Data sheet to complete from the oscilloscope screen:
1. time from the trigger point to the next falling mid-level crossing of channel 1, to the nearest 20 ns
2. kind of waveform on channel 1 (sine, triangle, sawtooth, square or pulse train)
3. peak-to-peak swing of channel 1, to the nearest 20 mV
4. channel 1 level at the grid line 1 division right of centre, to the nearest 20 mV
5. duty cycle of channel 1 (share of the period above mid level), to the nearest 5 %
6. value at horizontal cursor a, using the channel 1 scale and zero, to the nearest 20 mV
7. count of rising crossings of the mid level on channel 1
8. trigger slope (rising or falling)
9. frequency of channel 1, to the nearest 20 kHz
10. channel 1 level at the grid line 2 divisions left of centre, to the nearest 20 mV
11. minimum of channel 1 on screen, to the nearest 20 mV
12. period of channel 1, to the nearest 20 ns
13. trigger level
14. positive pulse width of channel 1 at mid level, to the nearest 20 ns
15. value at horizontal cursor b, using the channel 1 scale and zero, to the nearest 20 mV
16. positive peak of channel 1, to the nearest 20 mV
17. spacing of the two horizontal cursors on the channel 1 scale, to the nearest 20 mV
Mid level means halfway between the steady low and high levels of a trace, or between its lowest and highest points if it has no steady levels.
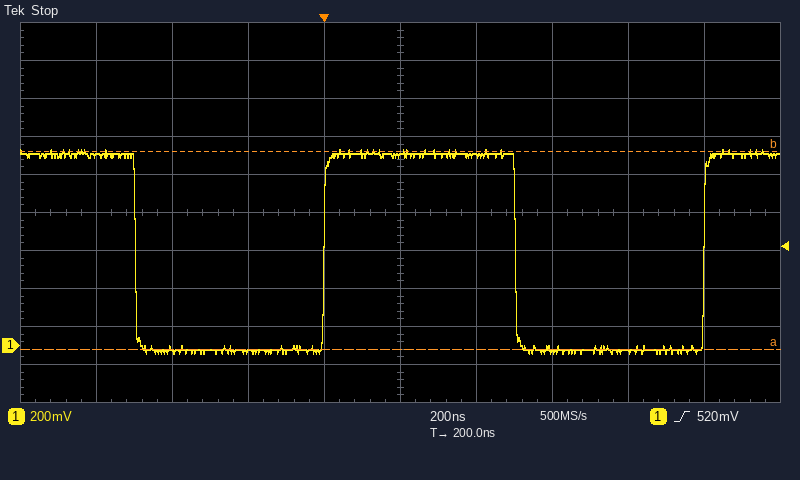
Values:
500 ns
square
1.08 V
1.00 V
50 %
-20 mV
2
rising
1.00 MHz
-40 mV
-40 mV
1.00 µs
520 mV
500 ns
1.02 V
1.04 V
1.04 V
